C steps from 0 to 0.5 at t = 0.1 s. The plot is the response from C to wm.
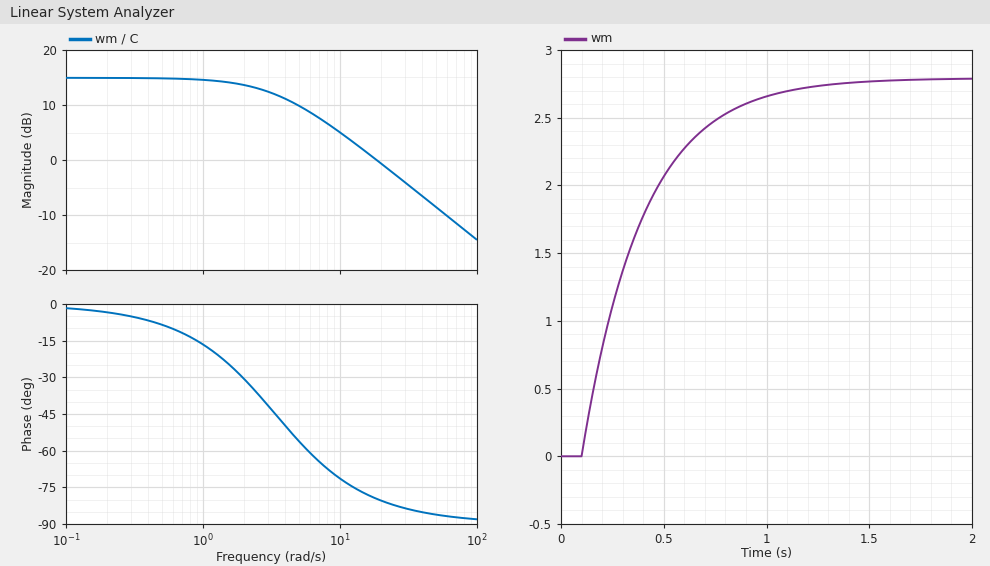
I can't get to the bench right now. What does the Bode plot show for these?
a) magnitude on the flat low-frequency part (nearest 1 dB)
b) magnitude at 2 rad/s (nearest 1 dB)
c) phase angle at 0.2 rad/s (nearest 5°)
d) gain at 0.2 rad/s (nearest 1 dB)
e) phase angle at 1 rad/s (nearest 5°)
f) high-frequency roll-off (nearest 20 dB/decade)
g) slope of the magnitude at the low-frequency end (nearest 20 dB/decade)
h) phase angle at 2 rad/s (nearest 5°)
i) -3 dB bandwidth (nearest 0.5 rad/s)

15 dB
14 dB
-5°
15 dB
-15°
-20 dB/decade
0 dB/decade
-30°
3.5 rad/s
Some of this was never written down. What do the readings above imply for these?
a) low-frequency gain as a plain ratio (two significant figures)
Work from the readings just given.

5.6
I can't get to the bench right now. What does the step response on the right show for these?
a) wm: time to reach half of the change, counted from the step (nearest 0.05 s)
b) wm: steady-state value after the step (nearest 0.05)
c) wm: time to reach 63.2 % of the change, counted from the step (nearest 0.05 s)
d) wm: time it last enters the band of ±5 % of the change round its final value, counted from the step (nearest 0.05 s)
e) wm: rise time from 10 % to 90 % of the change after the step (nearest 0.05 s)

0.20 s
2.80
0.30 s
0.90 s
0.65 s
